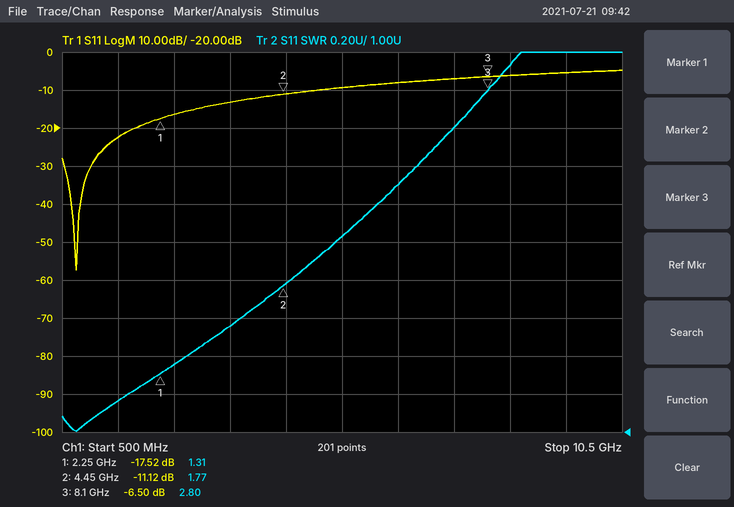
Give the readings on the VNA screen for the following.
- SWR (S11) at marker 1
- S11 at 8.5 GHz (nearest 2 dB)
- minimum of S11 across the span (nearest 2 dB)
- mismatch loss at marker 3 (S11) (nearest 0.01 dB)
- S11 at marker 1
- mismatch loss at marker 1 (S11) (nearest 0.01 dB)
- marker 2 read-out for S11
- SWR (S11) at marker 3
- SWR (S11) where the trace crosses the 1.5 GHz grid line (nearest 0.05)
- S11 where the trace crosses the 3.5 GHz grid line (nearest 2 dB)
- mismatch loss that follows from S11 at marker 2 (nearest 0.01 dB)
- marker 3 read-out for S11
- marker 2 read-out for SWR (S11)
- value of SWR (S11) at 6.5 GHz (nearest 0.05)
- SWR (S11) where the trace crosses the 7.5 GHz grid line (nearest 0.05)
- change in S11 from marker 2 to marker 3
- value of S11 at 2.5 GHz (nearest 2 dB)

1.31
-6 dB
-58 dB
1.10 dB
-17.52 dB
0.08 dB
-11.12 dB
2.80
1.15
-14 dB
0.35 dB
-6.50 dB
1.77
2.30
2.60
4.62 dB
-16 dB
